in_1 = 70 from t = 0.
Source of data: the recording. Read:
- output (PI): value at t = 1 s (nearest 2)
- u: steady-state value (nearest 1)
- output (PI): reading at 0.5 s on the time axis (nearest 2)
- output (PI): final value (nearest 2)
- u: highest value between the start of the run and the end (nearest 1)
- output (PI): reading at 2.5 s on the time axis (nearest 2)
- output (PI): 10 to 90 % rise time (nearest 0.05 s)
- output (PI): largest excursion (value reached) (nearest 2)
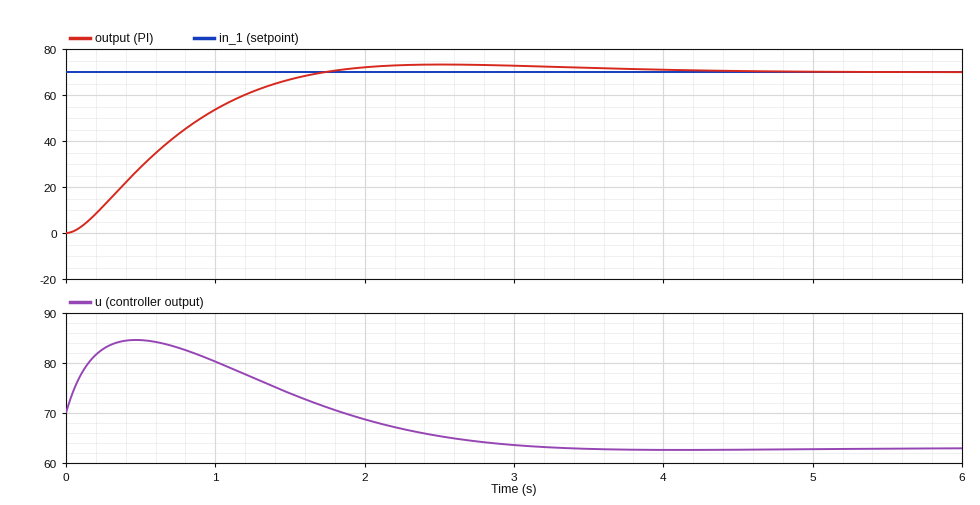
54
63
28
70
85
74
1.15 s
74
